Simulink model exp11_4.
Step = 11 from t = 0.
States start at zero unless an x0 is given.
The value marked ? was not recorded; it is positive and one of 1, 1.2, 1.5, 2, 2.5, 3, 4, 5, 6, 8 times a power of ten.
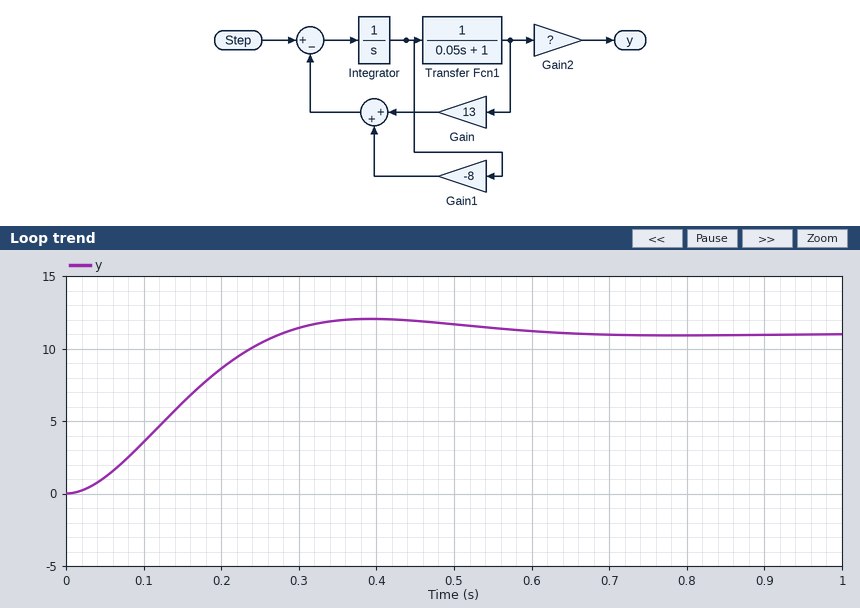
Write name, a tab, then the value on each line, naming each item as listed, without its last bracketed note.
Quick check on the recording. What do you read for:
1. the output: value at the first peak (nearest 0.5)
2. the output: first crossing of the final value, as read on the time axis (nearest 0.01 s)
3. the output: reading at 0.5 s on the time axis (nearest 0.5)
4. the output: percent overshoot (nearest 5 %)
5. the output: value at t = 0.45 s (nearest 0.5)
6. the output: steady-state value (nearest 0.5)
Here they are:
the output: value at the first peak	12.0
the output: first crossing of the final value, as read on the time axis	0.28 s
the output: reading at 0.5 s on the time axis	11.5
the output: percent overshoot	10 %
the output: value at t = 0.45 s	12.0
the output: steady-state value	11.0
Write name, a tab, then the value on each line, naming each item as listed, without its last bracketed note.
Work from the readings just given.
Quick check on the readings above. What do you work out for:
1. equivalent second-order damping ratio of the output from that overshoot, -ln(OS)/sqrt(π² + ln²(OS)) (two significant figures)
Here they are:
equivalent second-order damping ratio of the output from that overshoot, -ln(OS)/sqrt(π² + ln²(OS))	0.59
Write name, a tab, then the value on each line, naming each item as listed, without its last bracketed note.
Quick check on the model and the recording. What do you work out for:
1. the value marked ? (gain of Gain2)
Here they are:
the value marked ?	5
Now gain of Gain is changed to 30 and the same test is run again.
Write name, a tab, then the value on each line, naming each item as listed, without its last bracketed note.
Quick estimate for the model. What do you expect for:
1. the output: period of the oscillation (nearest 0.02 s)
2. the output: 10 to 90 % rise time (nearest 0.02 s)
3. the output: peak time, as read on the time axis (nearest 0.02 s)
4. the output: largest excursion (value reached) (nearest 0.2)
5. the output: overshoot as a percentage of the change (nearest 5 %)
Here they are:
the output: period of the oscillation	0.32 s
the output: 10 to 90 % rise time	0.06 s
the output: peak time, as read on the time axis	0.16 s
the output: largest excursion (value reached)	3.4
the output: overshoot as a percentage of the change	40 %
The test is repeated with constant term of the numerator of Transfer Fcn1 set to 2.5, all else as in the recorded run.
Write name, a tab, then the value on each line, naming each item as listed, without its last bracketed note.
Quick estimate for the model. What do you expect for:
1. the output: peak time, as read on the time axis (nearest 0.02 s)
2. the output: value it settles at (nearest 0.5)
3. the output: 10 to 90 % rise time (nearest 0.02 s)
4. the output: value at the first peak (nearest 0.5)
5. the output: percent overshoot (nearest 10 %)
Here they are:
the output: peak time, as read on the time axis	0.14 s
the output: value it settles at	5.5
the output: 10 to 90 % rise time	0.06 s
the output: value at the first peak	8.0
the output: percent overshoot	40 %
